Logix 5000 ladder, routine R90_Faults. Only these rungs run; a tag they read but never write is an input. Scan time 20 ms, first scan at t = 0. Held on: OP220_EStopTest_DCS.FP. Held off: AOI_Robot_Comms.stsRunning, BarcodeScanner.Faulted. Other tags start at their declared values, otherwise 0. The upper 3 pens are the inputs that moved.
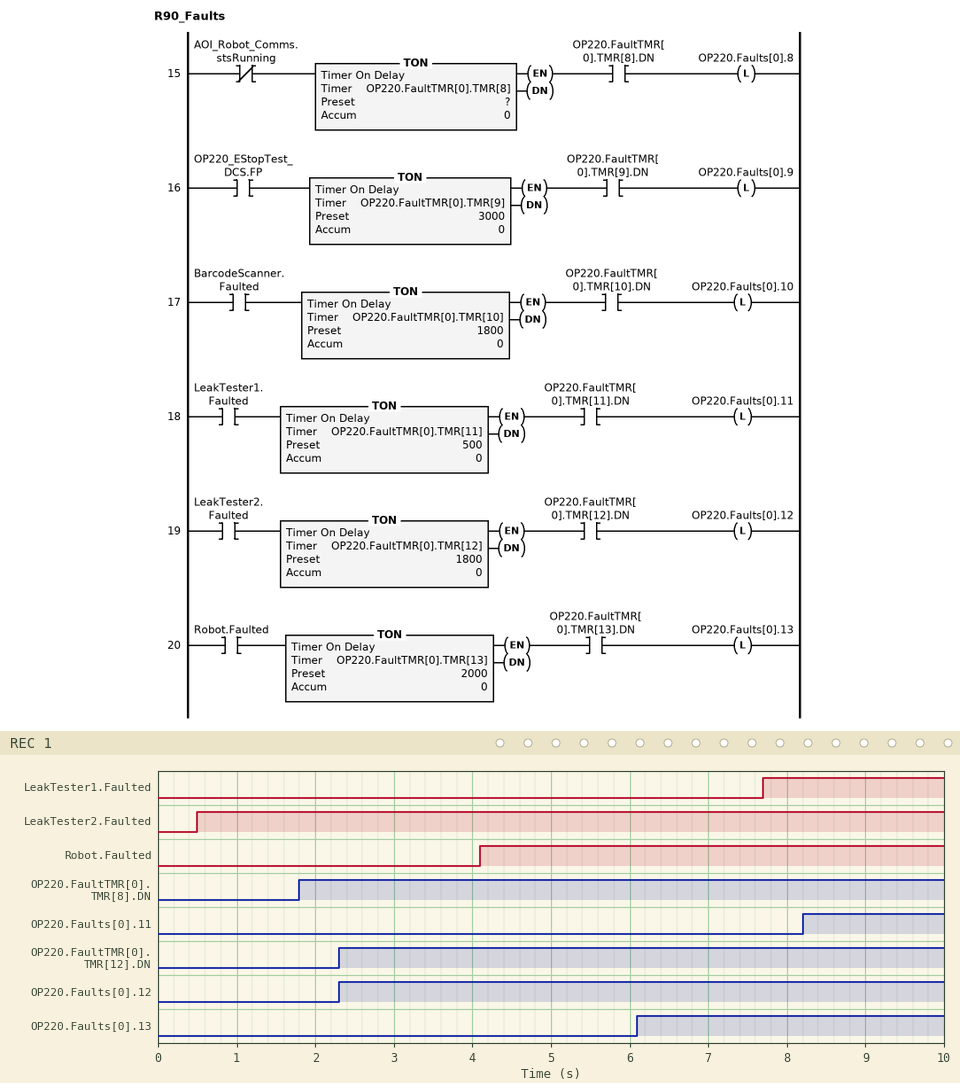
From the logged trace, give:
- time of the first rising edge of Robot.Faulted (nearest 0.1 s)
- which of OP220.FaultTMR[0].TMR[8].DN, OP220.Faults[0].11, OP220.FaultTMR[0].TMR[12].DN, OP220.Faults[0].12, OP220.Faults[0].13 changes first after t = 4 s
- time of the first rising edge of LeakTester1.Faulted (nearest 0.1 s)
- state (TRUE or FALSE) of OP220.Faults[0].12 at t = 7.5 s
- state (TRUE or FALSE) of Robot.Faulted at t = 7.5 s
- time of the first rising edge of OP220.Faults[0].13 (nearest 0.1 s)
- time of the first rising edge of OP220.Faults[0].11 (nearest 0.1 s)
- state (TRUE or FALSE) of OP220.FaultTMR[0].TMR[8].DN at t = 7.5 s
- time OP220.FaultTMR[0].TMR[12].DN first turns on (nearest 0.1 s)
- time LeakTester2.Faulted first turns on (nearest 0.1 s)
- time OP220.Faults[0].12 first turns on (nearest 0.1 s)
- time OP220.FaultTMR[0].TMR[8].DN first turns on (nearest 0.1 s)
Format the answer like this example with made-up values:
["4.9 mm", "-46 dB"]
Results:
["4.1 s", "OP220.Faults[0].13", "7.7 s", "TRUE", "TRUE", "6.1 s", "8.2 s", "TRUE", "2.3 s", "0.5 s", "2.3 s", "1.8 s"]
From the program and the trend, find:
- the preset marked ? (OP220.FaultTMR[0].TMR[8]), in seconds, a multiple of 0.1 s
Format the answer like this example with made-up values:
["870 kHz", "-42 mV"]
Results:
["1.8 s"]
